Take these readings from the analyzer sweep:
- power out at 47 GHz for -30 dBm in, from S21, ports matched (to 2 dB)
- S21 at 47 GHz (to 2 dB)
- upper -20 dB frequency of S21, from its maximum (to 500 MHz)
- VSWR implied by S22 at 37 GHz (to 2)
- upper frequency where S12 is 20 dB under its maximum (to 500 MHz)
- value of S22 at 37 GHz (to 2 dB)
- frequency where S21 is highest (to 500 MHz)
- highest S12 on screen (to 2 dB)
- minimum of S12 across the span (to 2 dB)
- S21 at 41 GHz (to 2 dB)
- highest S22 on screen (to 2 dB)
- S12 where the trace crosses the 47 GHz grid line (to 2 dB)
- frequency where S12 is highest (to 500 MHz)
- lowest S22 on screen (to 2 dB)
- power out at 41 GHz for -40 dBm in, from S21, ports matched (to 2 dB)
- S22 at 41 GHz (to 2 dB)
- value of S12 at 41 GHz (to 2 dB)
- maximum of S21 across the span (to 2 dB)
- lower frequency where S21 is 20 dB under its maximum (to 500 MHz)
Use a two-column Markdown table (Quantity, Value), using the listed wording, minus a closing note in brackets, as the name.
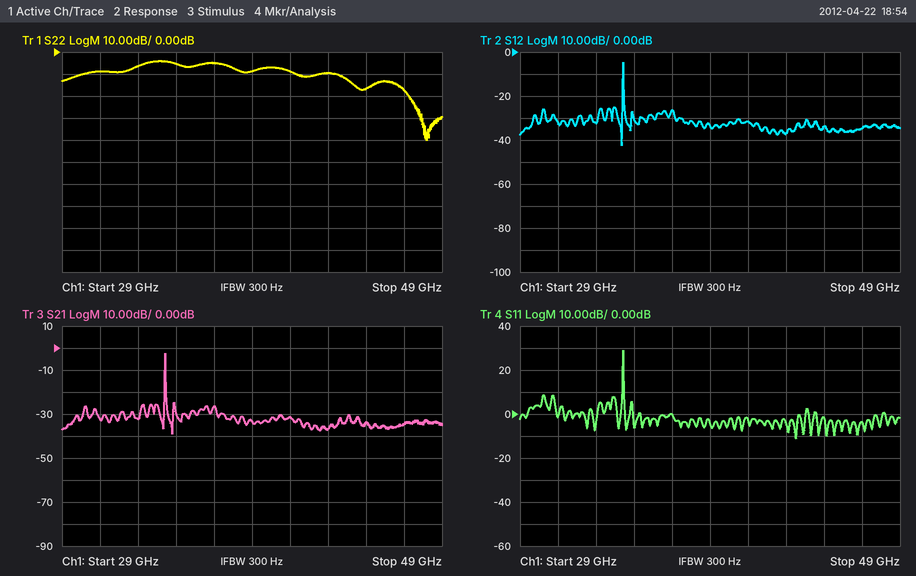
| Quantity | Value |
|---|---|
| power out at 47 GHz for -30 dBm in, from S21, ports matched | -64 dBm |
| S21 at 47 GHz | -34 dB |
| upper -20 dB frequency of S21, from its maximum | 34.5 GHz |
| VSWR implied by S22 at 37 GHz | 4 |
| upper frequency where S12 is 20 dB under its maximum | 34.5 GHz |
| value of S22 at 37 GHz | -4 dB |
| frequency where S21 is highest | 34.5 GHz |
| highest S12 on screen | -4 dB |
| minimum of S12 across the span | -42 dB |
| S21 at 41 GHz | -32 dB |
| highest S22 on screen | -4 dB |
| S12 where the trace crosses the 47 GHz grid line | -34 dB |
| frequency where S12 is highest | 34.5 GHz |
| lowest S22 on screen | -40 dB |
| power out at 41 GHz for -40 dBm in, from S21, ports matched | -72 dBm |
| S22 at 41 GHz | -8 dB |
| value of S12 at 41 GHz | -32 dB |
| maximum of S21 across the span | -2 dB |
| lower frequency where S21 is 20 dB under its maximum | 34.5 GHz |
